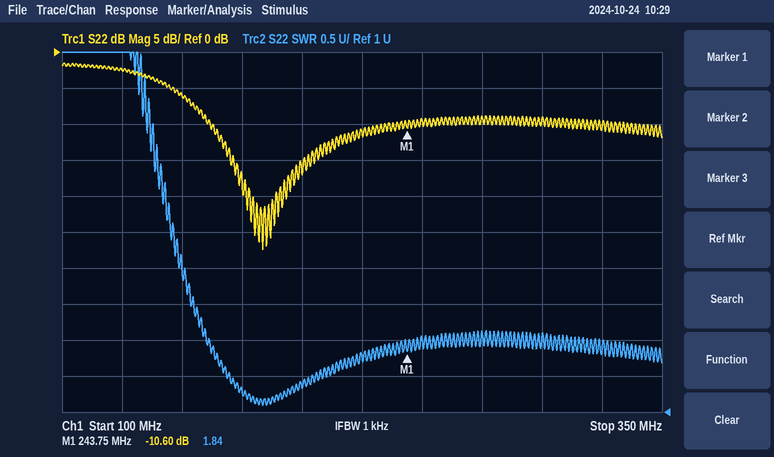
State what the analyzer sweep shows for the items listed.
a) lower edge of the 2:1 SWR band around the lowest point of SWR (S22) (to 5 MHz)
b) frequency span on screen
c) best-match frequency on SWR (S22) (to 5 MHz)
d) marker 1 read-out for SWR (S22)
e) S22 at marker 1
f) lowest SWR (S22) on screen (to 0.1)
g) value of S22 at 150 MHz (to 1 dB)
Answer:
160 MHz
250 MHz
185 MHz
1.84
-10.60 dB
1.1
-6 dB
